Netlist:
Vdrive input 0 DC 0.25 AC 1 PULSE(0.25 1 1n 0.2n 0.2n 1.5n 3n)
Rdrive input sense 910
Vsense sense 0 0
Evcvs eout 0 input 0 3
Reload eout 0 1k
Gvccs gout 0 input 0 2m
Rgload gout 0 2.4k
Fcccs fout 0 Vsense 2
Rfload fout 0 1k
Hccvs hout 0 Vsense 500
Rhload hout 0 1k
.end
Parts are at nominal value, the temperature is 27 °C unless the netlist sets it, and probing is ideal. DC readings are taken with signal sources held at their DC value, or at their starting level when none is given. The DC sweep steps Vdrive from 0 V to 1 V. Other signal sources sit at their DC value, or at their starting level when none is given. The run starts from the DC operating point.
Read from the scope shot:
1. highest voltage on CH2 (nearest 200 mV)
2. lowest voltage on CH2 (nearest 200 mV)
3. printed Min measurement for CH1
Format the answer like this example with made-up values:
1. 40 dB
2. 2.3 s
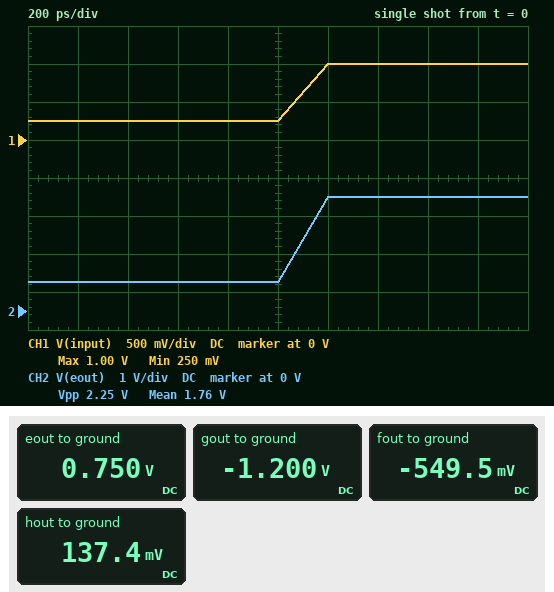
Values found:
1. 3.0 V
2. 800 mV
3. 250 mV
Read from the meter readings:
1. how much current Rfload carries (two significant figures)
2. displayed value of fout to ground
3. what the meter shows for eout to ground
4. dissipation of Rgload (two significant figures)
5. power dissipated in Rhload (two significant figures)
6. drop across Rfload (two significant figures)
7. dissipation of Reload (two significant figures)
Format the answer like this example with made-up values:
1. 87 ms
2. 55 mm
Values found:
1. 550 µA
2. -549.5 mV
3. 0.750 V
4. 600 µW
5. 19 µW
6. 550 mV
7. 560 µW
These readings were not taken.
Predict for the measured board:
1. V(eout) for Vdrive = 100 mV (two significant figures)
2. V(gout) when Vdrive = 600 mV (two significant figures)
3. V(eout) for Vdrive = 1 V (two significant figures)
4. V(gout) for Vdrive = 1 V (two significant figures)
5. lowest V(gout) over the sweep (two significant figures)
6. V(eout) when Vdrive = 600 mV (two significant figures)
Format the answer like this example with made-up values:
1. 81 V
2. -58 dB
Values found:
1. 300 mV
2. -2.9 V
3. 3.0 V
4. -4.8 V
5. -4.8 V
6. 1.8 V
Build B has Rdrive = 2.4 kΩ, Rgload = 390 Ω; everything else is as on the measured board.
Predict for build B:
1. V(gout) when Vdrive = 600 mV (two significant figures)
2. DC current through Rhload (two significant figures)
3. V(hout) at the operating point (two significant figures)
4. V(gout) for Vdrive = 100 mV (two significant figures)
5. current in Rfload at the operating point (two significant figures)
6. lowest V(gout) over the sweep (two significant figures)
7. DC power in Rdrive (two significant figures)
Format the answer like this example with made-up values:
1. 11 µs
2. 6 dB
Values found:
1. -470 mV
2. 52 µA
3. 52 mV
4. -78 mV
5. 210 µA
6. -780 mV
7. 26 µW
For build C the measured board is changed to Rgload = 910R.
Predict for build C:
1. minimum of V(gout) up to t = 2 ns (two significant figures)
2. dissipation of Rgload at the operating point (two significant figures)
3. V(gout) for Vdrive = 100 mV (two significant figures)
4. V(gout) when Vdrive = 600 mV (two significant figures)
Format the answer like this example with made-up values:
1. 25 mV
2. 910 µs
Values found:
1. -1.8 V
2. 230 µW
3. -180 mV
4. -1.1 V
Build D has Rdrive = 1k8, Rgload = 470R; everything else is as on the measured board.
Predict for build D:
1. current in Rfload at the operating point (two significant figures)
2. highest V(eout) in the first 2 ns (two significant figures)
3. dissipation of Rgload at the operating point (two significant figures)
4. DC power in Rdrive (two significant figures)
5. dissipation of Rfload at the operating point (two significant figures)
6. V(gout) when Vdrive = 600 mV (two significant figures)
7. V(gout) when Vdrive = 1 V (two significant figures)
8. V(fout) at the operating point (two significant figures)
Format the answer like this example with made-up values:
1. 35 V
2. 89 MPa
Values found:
1. 280 µA
2. 3.0 V
3. 120 µW
4. 35 µW
5. 77 µW
6. -560 mV
7. -940 mV
8. -280 mV
